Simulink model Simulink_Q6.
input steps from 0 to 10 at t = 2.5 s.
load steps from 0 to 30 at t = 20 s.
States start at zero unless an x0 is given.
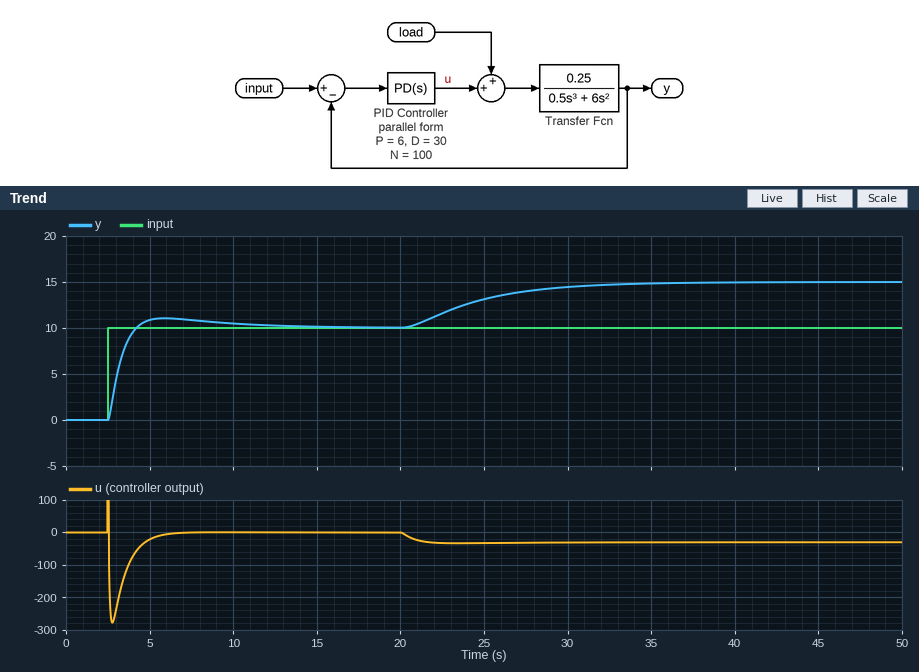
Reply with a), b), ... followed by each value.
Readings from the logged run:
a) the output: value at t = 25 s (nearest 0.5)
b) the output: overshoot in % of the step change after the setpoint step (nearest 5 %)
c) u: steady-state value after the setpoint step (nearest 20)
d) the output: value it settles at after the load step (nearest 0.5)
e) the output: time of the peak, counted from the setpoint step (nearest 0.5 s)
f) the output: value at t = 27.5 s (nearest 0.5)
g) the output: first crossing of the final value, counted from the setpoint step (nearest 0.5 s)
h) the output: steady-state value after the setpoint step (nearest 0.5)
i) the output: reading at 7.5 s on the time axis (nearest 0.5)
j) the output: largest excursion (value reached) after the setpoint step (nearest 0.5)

a) 13.0
b) 10 %
c) 0
d) 15.0
e) 3.5 s
f) 14.0
g) 1.5 s
h) 10.0
i) 11.0
j) 11.0
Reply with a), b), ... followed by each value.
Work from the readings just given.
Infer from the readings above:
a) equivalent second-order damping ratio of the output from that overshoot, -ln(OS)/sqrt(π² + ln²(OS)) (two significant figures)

a) 0.59
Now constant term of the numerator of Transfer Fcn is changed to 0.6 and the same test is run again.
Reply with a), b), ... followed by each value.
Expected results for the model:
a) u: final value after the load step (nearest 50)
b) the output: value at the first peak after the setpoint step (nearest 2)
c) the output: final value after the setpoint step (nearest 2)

a) -50
b) 10
c) 10
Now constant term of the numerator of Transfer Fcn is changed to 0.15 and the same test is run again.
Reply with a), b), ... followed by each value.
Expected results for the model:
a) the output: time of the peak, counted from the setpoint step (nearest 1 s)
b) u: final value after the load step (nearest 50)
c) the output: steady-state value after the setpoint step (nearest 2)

a) 5 s
b) -50
c) 10
